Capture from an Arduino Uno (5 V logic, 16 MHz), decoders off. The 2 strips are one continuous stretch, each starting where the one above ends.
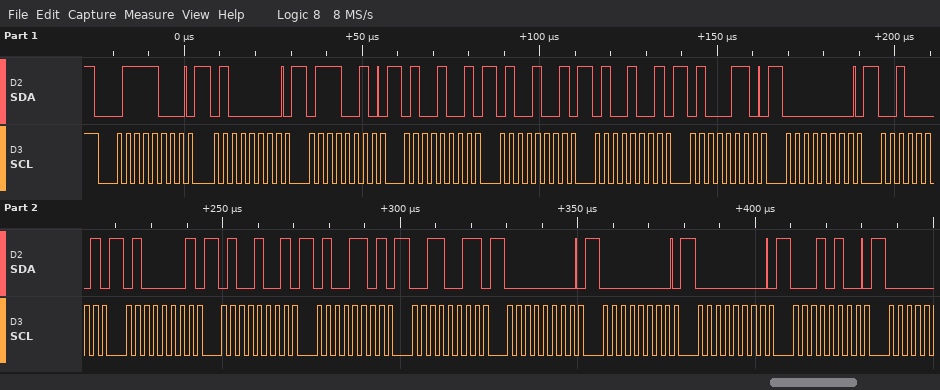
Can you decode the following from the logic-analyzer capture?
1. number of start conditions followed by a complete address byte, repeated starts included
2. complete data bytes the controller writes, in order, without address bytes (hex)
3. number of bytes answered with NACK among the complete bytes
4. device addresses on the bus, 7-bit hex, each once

1
40 72 49 49 49 46 00 21 41 49 4D 33 00 00 00 14
0
0x3C
